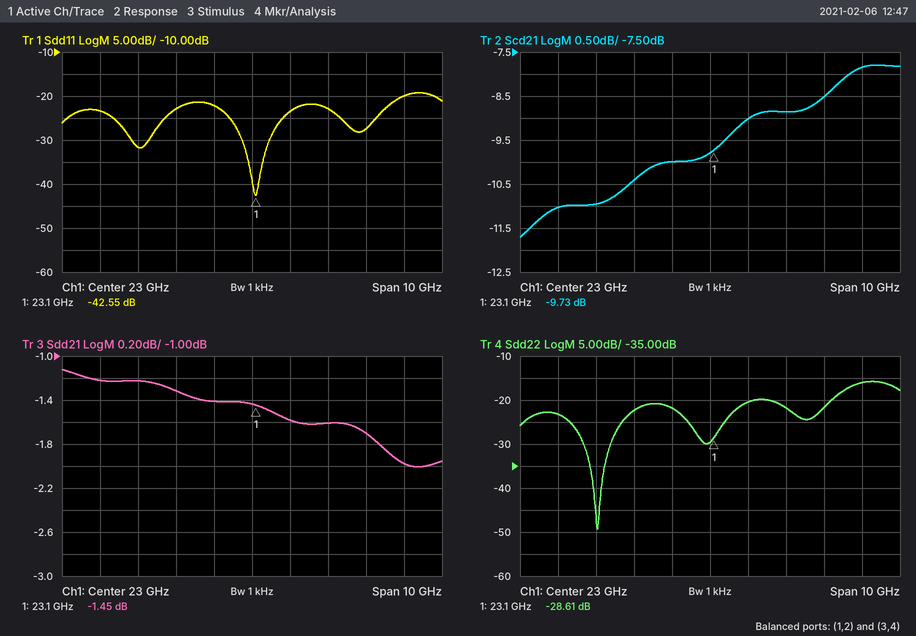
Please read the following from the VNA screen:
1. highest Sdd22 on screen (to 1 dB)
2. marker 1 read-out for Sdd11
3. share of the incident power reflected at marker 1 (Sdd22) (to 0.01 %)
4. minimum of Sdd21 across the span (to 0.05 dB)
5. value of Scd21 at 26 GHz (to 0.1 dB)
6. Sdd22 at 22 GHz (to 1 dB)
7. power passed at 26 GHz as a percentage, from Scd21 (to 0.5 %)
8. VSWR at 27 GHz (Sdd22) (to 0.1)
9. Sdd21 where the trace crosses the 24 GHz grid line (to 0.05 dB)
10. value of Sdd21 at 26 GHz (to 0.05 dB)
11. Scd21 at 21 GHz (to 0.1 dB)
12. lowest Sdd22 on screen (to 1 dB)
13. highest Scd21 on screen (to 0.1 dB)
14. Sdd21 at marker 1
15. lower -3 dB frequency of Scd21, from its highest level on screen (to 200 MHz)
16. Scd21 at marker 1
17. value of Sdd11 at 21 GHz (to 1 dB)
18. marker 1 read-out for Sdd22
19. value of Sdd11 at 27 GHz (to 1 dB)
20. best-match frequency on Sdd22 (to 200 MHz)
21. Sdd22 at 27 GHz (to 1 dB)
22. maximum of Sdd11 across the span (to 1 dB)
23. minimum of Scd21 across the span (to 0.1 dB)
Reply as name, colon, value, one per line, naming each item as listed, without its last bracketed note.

highest Sdd22 on screen: -16 dB
marker 1 read-out for Sdd11: -42.55 dB
share of the incident power reflected at marker 1 (Sdd22): 0.14 %
minimum of Sdd21 across the span: -2.00 dB
value of Scd21 at 26 GHz: -8.5 dB
Sdd22 at 22 GHz: -22 dB
power passed at 26 GHz as a percentage, from Scd21: 14.0 %
VSWR at 27 GHz (Sdd22): 1.4
Sdd21 where the trace crosses the 24 GHz grid line: -1.60 dB
value of Sdd21 at 26 GHz: -1.70 dB
Scd21 at 21 GHz: -10.4 dB
lowest Sdd22 on screen: -49 dB
highest Scd21 on screen: -7.8 dB
Sdd21 at marker 1: -1.45 dB
lower -3 dB frequency of Scd21, from its highest level on screen: 20.4 GHz
Scd21 at marker 1: -9.73 dB
value of Sdd11 at 21 GHz: -23 dB
marker 1 read-out for Sdd22: -28.61 dB
value of Sdd11 at 27 GHz: -20 dB
best-match frequency on Sdd22: 20.0 GHz
Sdd22 at 27 GHz: -16 dB
maximum of Sdd11 across the span: -19 dB
minimum of Scd21 across the span: -11.7 dB
